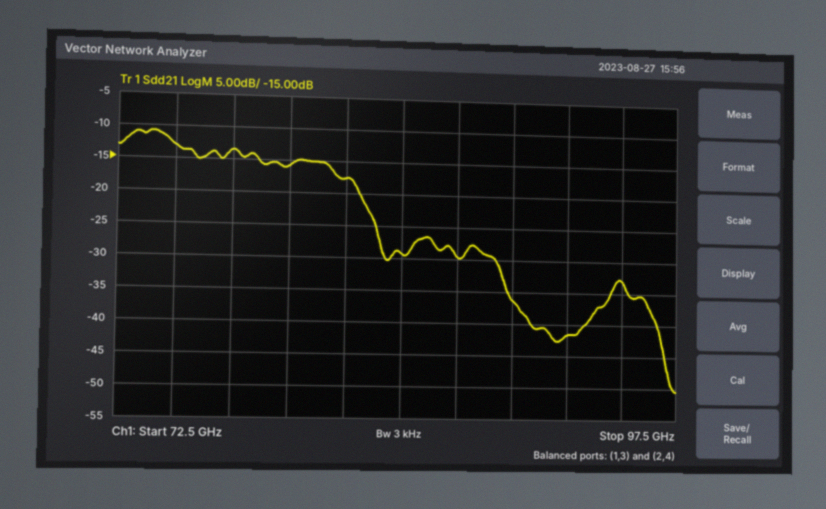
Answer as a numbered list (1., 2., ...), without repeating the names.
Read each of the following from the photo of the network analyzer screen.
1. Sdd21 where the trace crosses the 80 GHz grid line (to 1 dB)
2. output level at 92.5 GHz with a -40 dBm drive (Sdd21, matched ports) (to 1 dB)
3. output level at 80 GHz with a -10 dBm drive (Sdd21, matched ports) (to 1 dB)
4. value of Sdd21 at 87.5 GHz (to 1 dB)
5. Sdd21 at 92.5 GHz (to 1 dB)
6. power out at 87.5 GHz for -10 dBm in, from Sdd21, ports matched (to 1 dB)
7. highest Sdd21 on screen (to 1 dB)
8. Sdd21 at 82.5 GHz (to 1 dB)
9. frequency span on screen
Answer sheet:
1. -16 dB
2. -82 dBm
3. -26 dBm
4. -30 dB
5. -42 dB
6. -40 dBm
7. -11 dB
8. -18 dB
9. 25 GHz
